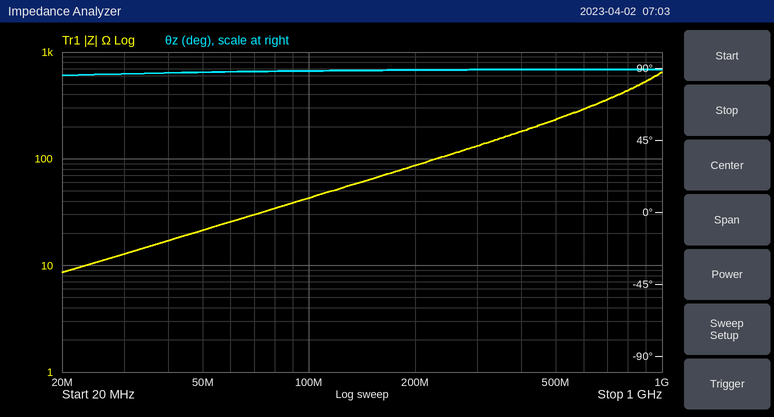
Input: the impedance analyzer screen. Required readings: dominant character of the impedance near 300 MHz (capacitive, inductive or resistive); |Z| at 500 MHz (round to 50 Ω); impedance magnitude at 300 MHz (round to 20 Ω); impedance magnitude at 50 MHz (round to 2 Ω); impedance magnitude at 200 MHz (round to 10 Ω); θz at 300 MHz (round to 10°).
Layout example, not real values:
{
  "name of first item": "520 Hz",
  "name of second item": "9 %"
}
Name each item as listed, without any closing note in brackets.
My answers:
{
  "dominant character of the impedance near 300 MHz": "inductive",
  "|Z| at 500 MHz": "250 Ω",
  "impedance magnitude at 300 MHz": "140 Ω",
  "impedance magnitude at 50 MHz": "22 Ω",
  "impedance magnitude at 200 MHz": "90 Ω",
  "θz at 300 MHz": "90°"
}
